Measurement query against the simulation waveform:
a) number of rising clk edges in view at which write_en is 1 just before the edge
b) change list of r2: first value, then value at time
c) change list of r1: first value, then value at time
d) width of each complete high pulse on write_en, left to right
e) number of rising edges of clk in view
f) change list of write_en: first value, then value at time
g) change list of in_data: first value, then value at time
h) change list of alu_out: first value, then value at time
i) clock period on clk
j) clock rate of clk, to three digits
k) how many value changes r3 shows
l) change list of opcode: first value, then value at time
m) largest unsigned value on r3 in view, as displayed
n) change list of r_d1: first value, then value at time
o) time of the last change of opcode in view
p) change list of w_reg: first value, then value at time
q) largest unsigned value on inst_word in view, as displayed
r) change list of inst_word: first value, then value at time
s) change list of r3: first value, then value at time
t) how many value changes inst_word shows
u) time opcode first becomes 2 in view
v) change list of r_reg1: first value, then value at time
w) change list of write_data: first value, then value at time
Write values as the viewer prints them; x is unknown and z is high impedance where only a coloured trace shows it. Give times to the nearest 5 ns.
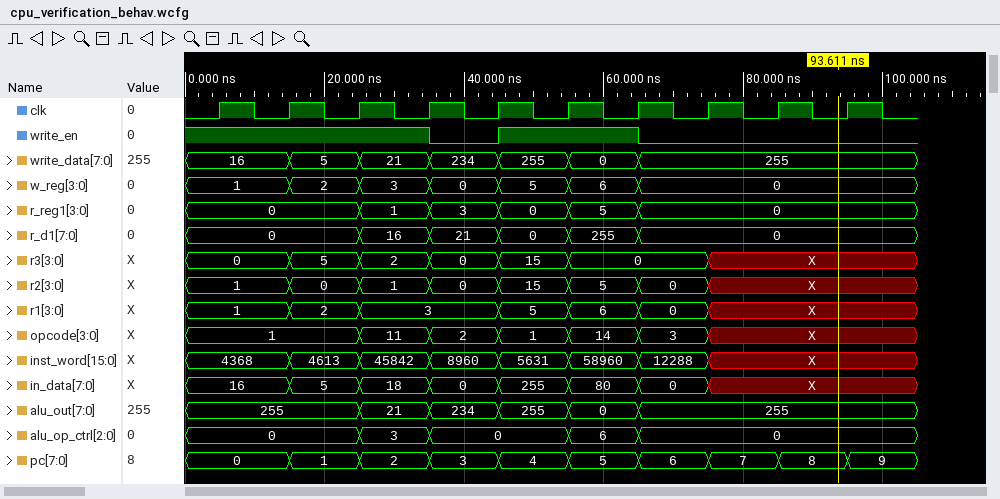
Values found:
6
1, 0 at 15 ns, 1 at 25 ns, 0 at 35 ns, 15 at 45 ns, 5 at 55 ns, 0 at 65 ns, X at 75 ns
1, 2 at 15 ns, 3 at 25 ns, 5 at 45 ns, 6 at 55 ns, 0 at 65 ns, X at 75 ns
20 ns
10
1, 0 at 35 ns, 1 at 45 ns, 0 at 65 ns
16, 5 at 15 ns, 18 at 25 ns, 0 at 35 ns, 255 at 45 ns, 80 at 55 ns, 0 at 65 ns, X at 75 ns
255, 21 at 25 ns, 234 at 35 ns, 255 at 45 ns, 0 at 55 ns, 255 at 65 ns
10 ns
100 MHz
6
1, 11 at 25 ns, 2 at 35 ns, 1 at 45 ns, 14 at 55 ns, 3 at 65 ns, X at 75 ns
15
0, 16 at 25 ns, 21 at 35 ns, 0 at 45 ns, 255 at 55 ns, 0 at 65 ns
75 ns
1, 2 at 15 ns, 3 at 25 ns, 0 at 35 ns, 5 at 45 ns, 6 at 55 ns, 0 at 65 ns
58960
4368, 4613 at 15 ns, 45842 at 25 ns, 8960 at 35 ns, 5631 at 45 ns, 58960 at 55 ns, 12288 at 65 ns, X at 75 ns
0, 5 at 15 ns, 2 at 25 ns, 0 at 35 ns, 15 at 45 ns, 0 at 55 ns, X at 75 ns
7
35 ns
0, 1 at 25 ns, 3 at 35 ns, 0 at 45 ns, 5 at 55 ns, 0 at 65 ns
16, 5 at 15 ns, 21 at 25 ns, 234 at 35 ns, 255 at 45 ns, 0 at 55 ns, 255 at 65 ns
